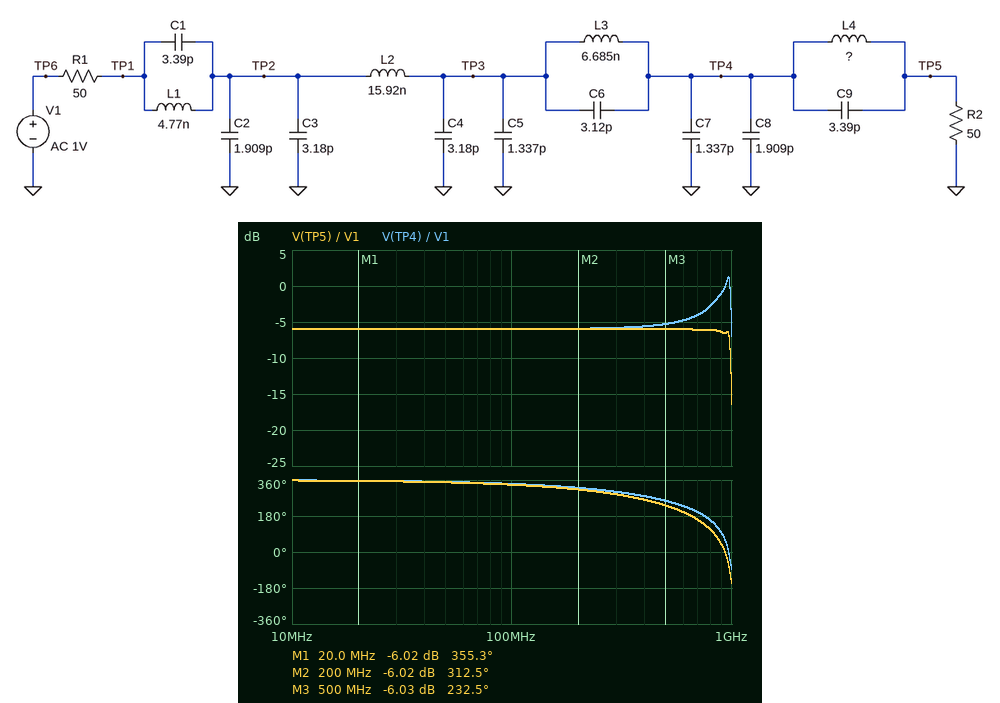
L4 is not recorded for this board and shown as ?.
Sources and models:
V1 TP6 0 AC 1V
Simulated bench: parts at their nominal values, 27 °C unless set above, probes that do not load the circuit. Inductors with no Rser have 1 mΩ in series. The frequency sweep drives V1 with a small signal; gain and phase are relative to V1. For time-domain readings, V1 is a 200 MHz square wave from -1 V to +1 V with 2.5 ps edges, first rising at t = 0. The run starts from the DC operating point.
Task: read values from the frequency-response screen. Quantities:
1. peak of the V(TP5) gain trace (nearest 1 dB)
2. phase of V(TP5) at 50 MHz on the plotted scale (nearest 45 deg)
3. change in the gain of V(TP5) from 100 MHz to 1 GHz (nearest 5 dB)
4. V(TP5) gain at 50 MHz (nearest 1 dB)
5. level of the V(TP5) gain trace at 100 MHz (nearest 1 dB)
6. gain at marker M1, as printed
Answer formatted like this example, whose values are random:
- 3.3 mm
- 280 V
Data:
- -6 dB
- 360 deg
- -10 dB
- -6 dB
- -6 dB
- -6.02 dB
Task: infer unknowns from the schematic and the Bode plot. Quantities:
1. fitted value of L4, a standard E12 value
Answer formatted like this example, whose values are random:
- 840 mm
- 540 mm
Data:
- 5.6 nH
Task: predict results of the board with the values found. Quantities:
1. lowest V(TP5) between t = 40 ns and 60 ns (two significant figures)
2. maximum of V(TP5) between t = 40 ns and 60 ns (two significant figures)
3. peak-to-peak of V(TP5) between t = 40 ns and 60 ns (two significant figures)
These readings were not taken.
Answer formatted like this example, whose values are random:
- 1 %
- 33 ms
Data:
- -630 mV
- 630 mV
- 1.3 V
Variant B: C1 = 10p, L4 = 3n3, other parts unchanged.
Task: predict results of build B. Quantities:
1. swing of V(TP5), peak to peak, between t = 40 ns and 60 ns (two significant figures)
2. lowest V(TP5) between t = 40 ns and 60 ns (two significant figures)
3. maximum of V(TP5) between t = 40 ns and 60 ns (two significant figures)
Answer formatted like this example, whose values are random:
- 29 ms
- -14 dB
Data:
- 1.4 V
- -690 mV
- 690 mV
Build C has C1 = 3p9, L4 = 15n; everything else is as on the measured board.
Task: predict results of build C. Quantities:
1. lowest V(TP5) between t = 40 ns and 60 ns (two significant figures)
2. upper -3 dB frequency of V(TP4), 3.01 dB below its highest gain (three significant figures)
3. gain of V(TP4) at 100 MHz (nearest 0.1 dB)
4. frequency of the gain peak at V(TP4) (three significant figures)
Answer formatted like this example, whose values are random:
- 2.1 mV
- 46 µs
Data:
- -640 mV
- 843 MHz
- -5.9 dB
- 646 MHz
